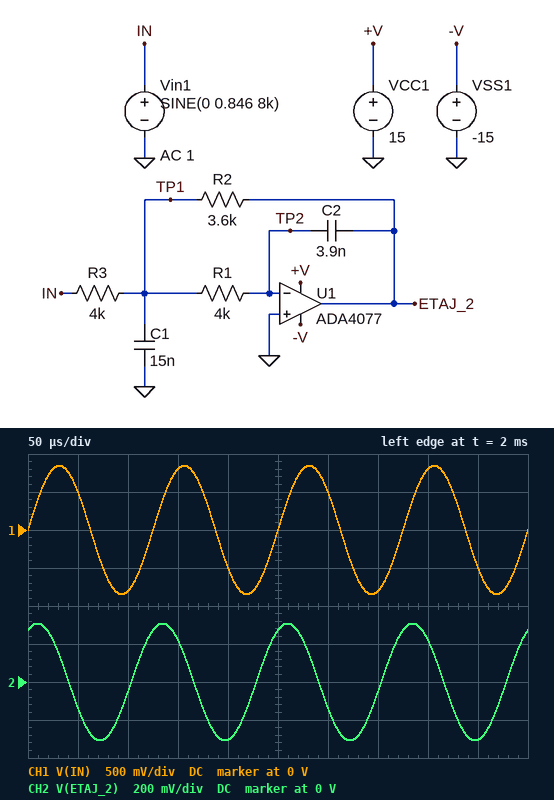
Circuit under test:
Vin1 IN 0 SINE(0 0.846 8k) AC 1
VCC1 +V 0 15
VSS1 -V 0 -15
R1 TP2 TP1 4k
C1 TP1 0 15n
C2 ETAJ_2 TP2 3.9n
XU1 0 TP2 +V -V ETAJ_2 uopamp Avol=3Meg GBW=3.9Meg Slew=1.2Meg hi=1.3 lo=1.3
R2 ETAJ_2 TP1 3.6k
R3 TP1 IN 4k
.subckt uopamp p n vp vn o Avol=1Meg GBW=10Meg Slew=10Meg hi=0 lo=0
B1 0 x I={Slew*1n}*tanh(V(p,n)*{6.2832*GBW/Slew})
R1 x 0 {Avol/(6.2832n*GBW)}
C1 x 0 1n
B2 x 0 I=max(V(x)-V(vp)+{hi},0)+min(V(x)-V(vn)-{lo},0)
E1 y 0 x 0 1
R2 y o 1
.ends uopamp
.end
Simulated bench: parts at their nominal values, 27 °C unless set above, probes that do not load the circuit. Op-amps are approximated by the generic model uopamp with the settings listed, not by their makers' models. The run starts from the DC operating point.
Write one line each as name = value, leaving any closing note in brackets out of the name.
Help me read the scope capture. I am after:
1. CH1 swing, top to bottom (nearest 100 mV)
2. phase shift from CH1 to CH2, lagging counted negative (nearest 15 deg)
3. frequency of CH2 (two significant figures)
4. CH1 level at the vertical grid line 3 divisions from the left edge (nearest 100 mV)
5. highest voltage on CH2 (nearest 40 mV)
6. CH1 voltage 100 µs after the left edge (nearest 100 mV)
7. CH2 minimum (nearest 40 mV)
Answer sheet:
CH1 swing, top to bottom = 1.7 V
phase shift from CH1 to CH2, lagging counted negative = 60 deg
frequency of CH2 = 8.0 kHz
CH1 level at the vertical grid line 3 divisions from the left edge = 800 mV
highest voltage on CH2 = 320 mV
CH1 voltage 100 µs after the left edge = -800 mV
CH2 minimum = -320 mV
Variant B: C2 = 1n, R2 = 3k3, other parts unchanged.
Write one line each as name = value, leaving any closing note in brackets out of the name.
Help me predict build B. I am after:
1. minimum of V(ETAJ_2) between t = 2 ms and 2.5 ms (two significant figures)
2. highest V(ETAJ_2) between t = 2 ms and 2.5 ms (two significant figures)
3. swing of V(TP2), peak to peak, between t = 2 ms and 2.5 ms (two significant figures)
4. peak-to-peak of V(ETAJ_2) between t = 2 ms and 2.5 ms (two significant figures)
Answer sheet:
minimum of V(ETAJ_2) between t = 2 ms and 2.5 ms = -960 mV
highest V(ETAJ_2) between t = 2 ms and 2.5 ms = 960 mV
swing of V(TP2), peak to peak, between t = 2 ms and 2.5 ms = 3.9 mV
peak-to-peak of V(ETAJ_2) between t = 2 ms and 2.5 ms = 1.9 V
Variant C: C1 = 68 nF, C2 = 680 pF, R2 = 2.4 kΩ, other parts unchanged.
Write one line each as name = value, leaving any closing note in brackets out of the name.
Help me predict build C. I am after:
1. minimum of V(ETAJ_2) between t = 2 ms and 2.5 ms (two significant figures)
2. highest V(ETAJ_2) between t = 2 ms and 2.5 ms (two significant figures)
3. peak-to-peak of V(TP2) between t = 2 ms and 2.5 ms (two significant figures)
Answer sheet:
minimum of V(ETAJ_2) between t = 2 ms and 2.5 ms = -1.5 V
highest V(ETAJ_2) between t = 2 ms and 2.5 ms = 1.5 V
peak-to-peak of V(TP2) between t = 2 ms and 2.5 ms = 6.3 mV
